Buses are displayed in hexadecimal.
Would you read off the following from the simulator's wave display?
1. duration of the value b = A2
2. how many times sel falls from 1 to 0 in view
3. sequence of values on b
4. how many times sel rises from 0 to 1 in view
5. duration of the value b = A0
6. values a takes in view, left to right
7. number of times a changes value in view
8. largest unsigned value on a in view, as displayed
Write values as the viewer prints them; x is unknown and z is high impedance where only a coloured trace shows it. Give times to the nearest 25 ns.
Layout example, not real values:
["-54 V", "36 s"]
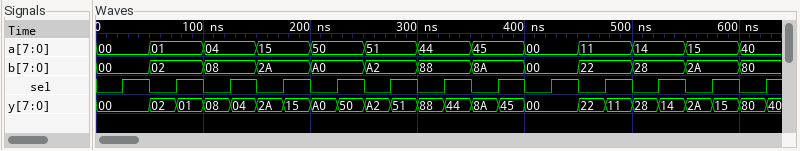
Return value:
["50 ns", "12", "00, 02, 08, 2A, A0, A2, 88, 8A, 00, 22, 28, 2A, 80", "13", "50 ns", "00, 01, 04, 15, 50, 51, 44, 45, 00, 11, 14, 15, 40", "12", "51"]
